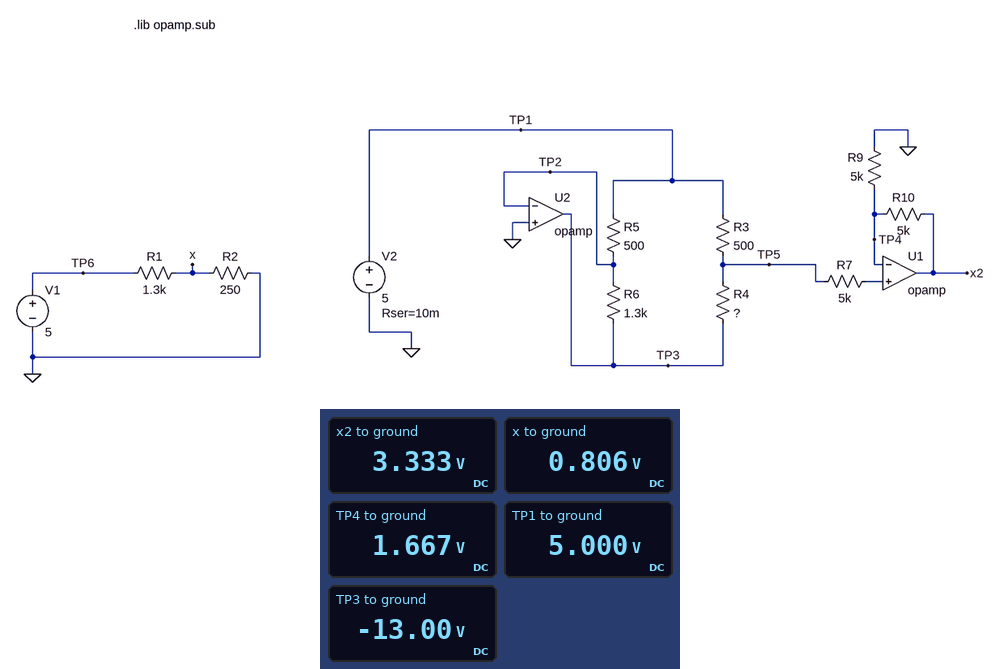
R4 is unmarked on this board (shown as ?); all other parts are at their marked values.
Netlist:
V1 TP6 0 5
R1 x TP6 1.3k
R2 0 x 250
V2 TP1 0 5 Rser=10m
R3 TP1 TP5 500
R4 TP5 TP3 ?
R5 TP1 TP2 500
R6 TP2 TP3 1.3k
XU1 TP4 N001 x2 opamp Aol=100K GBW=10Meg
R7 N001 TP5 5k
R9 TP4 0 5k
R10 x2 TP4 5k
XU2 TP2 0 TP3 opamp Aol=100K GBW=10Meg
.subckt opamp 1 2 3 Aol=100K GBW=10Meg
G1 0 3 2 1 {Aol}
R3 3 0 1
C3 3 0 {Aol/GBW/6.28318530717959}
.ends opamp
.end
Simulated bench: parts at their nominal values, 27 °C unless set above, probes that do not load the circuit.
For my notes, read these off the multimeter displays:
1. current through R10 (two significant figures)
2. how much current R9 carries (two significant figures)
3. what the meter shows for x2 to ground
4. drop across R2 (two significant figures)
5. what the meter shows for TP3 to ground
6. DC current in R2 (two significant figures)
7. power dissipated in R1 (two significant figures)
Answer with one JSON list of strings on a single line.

["330 µA", "330 µA", "3.333 V", "810 mV", "-13.00 V", "3.2 mA", "14 mW"]
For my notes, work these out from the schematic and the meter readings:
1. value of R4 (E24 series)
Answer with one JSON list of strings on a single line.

["2.2 kΩ"]
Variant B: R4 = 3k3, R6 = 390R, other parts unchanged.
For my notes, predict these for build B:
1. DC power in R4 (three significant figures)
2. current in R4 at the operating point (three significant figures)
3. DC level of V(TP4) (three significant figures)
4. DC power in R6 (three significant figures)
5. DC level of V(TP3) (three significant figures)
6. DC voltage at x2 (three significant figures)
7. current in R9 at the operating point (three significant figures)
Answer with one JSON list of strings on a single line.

["18.1 mW", "2.34 mA", "3.83 V", "39.0 mW", "-3.90 V", "7.66 V", "766 µA"]
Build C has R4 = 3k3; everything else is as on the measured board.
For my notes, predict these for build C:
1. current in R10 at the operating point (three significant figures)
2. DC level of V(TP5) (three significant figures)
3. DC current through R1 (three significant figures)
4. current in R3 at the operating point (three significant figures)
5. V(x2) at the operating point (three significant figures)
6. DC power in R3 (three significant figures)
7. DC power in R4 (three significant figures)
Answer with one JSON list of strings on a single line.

["526 µA", "2.63 V", "3.23 mA", "4.74 mA", "5.26 V", "11.2 mW", "74.0 mW"]
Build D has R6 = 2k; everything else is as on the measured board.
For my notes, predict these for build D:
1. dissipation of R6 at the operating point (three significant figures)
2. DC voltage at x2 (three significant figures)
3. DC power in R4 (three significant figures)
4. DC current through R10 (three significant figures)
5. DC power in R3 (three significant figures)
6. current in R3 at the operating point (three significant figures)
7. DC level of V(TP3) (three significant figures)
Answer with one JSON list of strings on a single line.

["200 mW", "741 mV", "189 mW", "74.1 µA", "42.9 mW", "9.26 mA", "-20.0 V"]
